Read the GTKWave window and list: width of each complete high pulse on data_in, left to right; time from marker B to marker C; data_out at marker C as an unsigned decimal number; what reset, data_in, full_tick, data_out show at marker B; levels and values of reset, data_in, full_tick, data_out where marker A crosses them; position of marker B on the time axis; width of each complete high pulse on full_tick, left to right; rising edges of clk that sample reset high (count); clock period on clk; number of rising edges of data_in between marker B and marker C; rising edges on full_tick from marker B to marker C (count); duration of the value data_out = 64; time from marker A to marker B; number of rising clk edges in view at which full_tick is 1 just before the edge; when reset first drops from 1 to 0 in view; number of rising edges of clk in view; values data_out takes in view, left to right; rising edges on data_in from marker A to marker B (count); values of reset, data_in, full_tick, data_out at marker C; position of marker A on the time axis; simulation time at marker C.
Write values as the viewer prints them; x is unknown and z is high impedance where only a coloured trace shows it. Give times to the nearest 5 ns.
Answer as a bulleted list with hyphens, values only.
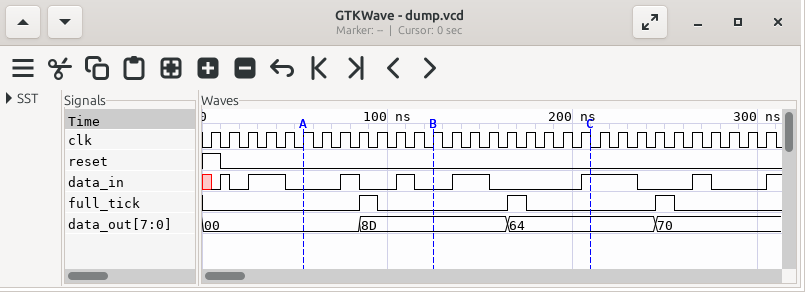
- 5 ns, 20 ns, 10 ns, 10 ns, 20 ns, 30 ns, 10 ns
- 85 ns
- 100
- reset=0, data_in=0, full_tick=0, data_out=8D
- reset=0, data_in=0, full_tick=0, data_out=00
- 125 ns
- 10 ns, 10 ns, 10 ns
- 1
- 10 ns
- 2
- 1
- 80 ns
- 70 ns
- 3
- 10 ns
- 31
- 00, 8D, 64, 70
- 2
- reset=0, data_in=1, full_tick=0, data_out=64
- 55 ns
- 210 ns
